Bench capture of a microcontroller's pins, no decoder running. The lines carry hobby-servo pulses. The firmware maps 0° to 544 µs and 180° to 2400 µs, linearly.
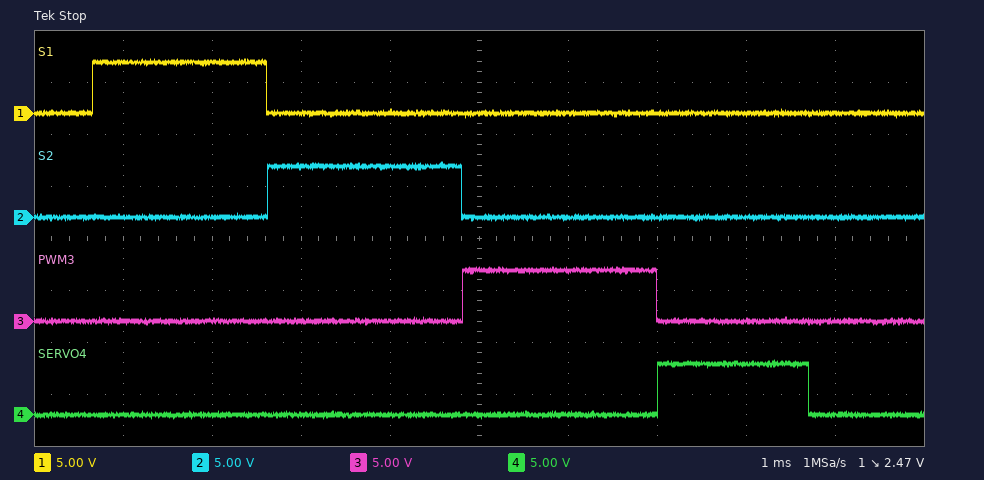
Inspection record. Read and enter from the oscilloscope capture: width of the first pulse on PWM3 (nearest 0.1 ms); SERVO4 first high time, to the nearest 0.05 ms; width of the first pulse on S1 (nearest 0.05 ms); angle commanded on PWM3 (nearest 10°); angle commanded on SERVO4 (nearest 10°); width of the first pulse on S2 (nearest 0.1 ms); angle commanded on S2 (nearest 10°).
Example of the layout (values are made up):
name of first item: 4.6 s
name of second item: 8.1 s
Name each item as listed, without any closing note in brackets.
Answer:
width of the first pulse on PWM3: 2.2 ms
SERVO4 first high time, to the nearest 0.05 ms: 1.70 ms
width of the first pulse on S1: 1.95 ms
angle commanded on PWM3: 160°
angle commanded on SERVO4: 110°
width of the first pulse on S2: 2.2 ms
angle commanded on S2: 160°
